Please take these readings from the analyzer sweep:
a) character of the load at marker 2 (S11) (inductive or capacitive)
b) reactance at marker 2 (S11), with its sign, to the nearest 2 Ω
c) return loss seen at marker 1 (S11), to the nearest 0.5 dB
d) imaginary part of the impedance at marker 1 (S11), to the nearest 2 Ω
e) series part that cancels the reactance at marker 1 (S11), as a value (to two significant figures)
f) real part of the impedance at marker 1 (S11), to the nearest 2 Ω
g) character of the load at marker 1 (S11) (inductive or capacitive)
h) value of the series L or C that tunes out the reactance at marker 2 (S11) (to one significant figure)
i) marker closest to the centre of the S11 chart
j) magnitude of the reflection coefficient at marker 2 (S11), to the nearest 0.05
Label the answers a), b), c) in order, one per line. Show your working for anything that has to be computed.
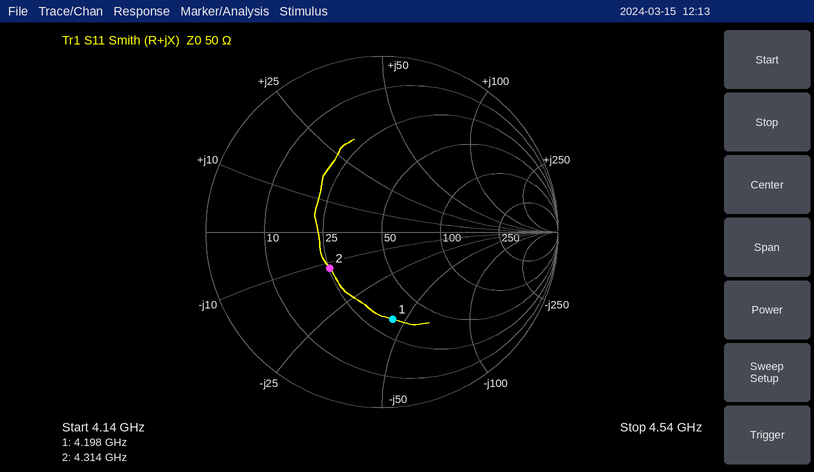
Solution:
a) capacitive
b) -12 Ω
c) 6.0 dB
d) -44 Ω
e) L = 44 Ω/(2π × 4.198 GHz) ≈ 1.7 nH
f) 34 Ω
g) capacitive
h) L = 12 Ω/(2π × 4.314 GHz) ≈ 443 pH, so 400 pH to one significant figure
i) marker 2
j) 0.35
